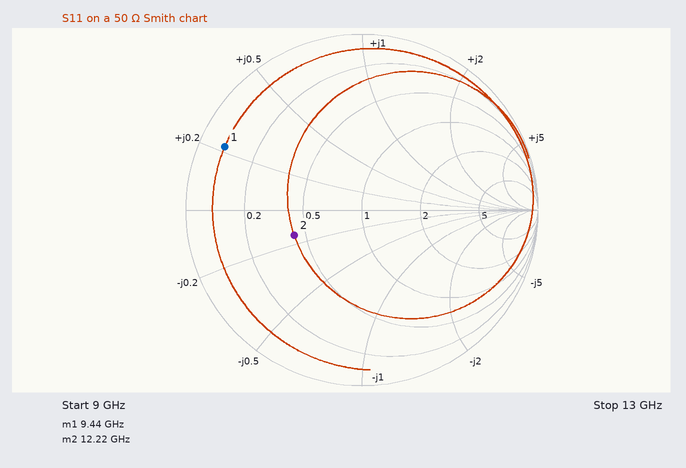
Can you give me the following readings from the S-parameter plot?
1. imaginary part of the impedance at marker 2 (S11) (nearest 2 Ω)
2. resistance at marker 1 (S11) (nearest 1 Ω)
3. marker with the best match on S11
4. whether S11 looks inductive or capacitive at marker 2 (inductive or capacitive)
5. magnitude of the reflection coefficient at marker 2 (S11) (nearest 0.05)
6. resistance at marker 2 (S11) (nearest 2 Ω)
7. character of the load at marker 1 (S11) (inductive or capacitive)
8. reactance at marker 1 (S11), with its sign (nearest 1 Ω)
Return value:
-8 Ω
4 Ω
marker 2
capacitive
0.40
22 Ω
inductive
+11 Ω
